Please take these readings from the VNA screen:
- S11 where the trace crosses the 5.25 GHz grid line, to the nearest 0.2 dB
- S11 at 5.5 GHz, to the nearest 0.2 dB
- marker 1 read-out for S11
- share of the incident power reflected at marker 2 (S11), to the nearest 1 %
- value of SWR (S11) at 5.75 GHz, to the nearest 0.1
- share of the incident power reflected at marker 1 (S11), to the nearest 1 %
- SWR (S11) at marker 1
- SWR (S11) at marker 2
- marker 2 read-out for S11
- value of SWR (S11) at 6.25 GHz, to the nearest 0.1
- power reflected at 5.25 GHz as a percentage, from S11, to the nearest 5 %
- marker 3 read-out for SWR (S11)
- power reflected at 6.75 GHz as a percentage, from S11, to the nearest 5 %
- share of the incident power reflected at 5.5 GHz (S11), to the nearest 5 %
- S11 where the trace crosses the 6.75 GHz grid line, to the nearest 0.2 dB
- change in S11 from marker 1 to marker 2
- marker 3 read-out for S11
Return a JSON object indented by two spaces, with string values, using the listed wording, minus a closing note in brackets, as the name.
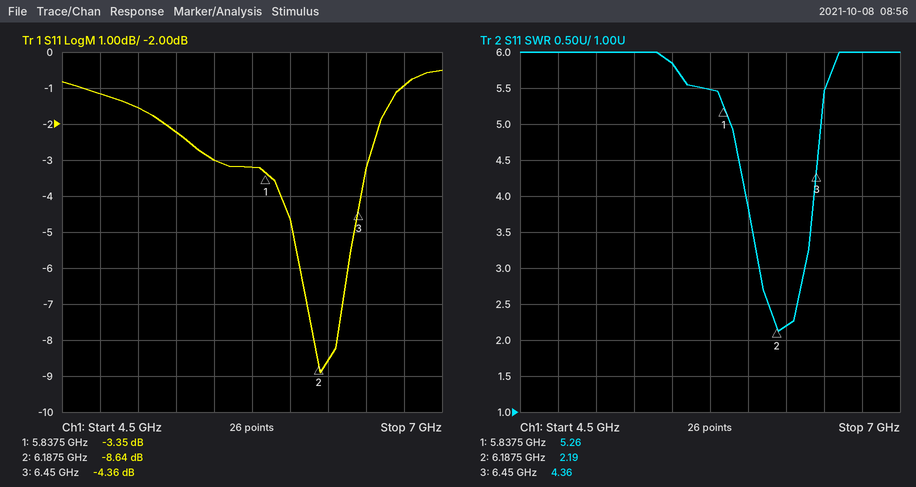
{
  "S11 where the trace crosses the 5.25 GHz grid line, to the nearest 0.2 dB": "-2.2 dB",
  "S11 at 5.5 GHz, to the nearest 0.2 dB": "-3.0 dB",
  "marker 1 read-out for S11": "-3.35 dB",
  "share of the incident power reflected at marker 2 (S11), to the nearest 1 %": "14 %",
  "value of SWR (S11) at 5.75 GHz, to the nearest 0.1": "5.5",
  "share of the incident power reflected at marker 1 (S11), to the nearest 1 %": "46 %",
  "SWR (S11) at marker 1": "5.26",
  "SWR (S11) at marker 2": "2.19",
  "marker 2 read-out for S11": "-8.64 dB",
  "value of SWR (S11) at 6.25 GHz, to the nearest 0.1": "2.2",
  "power reflected at 5.25 GHz as a percentage, from S11, to the nearest 5 %": "60 %",
  "marker 3 read-out for SWR": "4.36",
  "power reflected at 6.75 GHz as a percentage, from S11, to the nearest 5 %": "80 %",
  "share of the incident power reflected at 5.5 GHz (S11), to the nearest 5 %": "50 %",
  "S11 where the trace crosses the 6.75 GHz grid line, to the nearest 0.2 dB": "-1.0 dB",
  "change in S11 from marker 1 to marker 2": "-5.29 dB",
  "marker 3 read-out for S11": "-4.36 dB"
}
